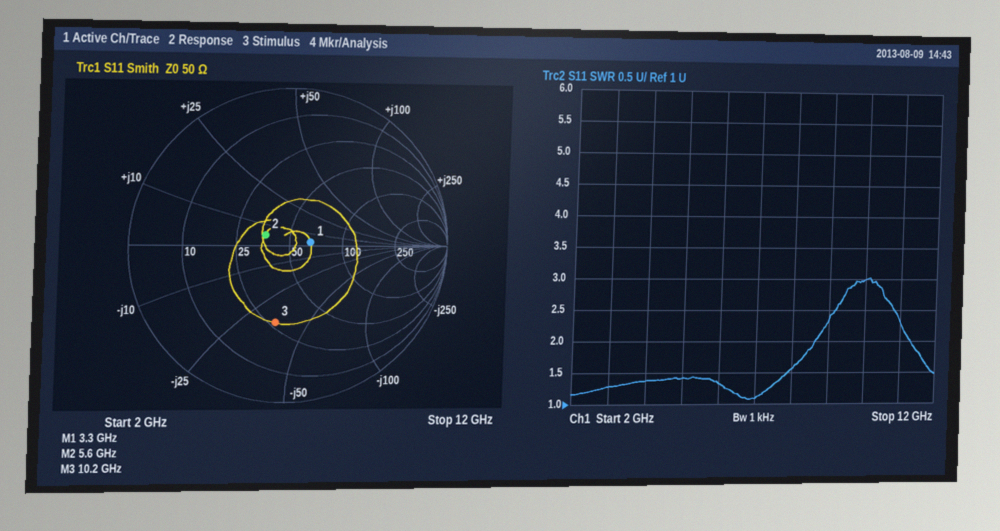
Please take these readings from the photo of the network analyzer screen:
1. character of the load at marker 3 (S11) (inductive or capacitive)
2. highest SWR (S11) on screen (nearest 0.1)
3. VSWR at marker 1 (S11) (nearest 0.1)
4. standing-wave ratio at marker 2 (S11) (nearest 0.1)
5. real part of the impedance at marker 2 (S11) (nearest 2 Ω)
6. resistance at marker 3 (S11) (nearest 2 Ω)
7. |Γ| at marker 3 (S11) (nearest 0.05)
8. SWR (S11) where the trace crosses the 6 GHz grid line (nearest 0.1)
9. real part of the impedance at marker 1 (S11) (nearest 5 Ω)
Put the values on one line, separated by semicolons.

capacitive; 3.0; 1.3; 1.4; 36 Ω; 28 Ω; 0.50; 1.3; 65 Ω
